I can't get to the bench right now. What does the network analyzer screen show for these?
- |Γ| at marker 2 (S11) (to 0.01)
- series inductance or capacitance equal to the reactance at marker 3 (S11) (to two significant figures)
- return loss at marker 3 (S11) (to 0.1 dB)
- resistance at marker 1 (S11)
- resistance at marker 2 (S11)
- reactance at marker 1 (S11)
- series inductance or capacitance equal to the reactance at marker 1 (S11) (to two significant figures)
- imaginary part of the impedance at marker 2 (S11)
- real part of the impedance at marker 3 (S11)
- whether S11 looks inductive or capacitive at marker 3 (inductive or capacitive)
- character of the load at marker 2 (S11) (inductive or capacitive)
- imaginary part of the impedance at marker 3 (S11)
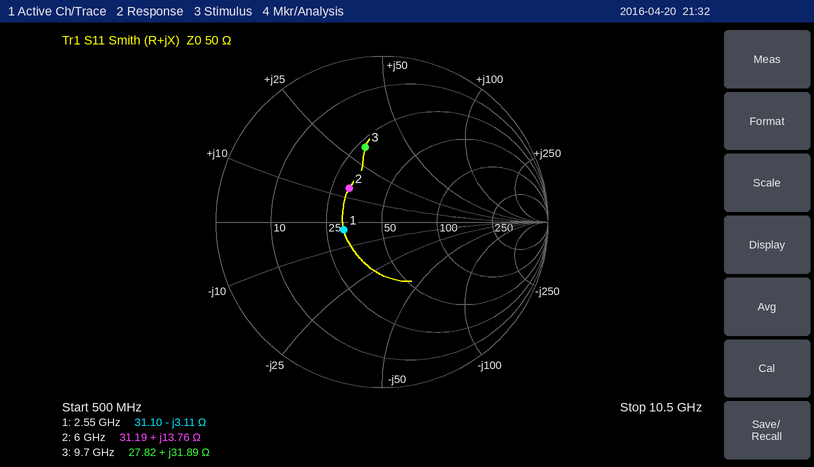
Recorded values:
0.28
520 pH
6.7 dB
31.10 Ω
31.19 Ω
-3.11 Ω
20 pF
+13.76 Ω
27.82 Ω
inductive
inductive
+31.89 Ω
